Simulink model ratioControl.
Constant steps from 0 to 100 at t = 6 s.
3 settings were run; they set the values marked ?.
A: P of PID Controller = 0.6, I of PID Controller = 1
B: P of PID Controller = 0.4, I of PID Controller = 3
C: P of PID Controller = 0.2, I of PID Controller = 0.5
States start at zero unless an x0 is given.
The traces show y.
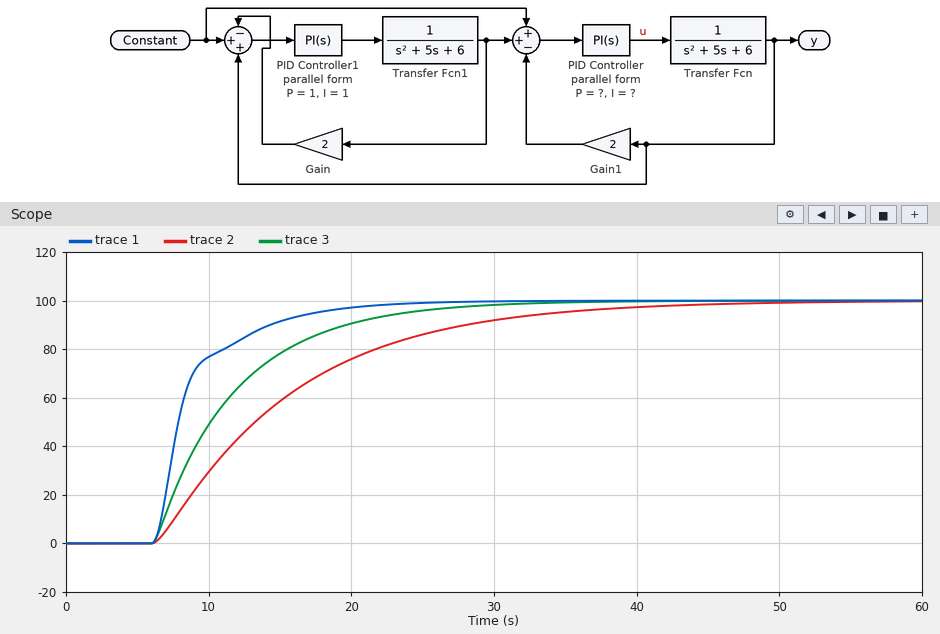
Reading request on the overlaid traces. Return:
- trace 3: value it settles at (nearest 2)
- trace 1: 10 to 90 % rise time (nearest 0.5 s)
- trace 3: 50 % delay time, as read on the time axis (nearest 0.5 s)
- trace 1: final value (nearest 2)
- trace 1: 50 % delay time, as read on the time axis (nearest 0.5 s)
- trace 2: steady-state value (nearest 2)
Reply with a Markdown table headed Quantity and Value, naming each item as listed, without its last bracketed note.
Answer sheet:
| Quantity | Value |
|---|---|
| trace 3: value it settles at | 100 |
| trace 1: 10 to 90 % rise time | 7.5 s |
| trace 3: 50 % delay time, as read on the time axis | 10.0 s |
| trace 1: final value | 100 |
| trace 1: 50 % delay time, as read on the time axis | 8.0 s |
| trace 2: steady-state value | 100 |
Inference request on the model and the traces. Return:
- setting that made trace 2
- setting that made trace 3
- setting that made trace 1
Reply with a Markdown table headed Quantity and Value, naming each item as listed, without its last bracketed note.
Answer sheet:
| Quantity | Value |
|---|---|
| setting that made trace 2 | C |
| setting that made trace 3 | A |
| setting that made trace 1 | B |
